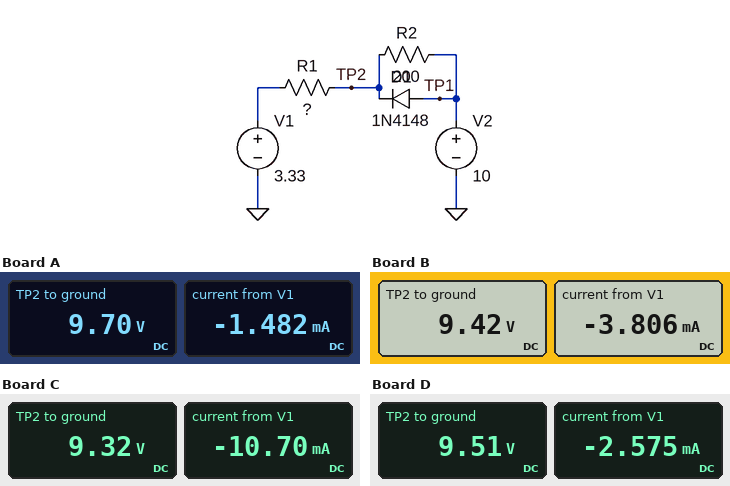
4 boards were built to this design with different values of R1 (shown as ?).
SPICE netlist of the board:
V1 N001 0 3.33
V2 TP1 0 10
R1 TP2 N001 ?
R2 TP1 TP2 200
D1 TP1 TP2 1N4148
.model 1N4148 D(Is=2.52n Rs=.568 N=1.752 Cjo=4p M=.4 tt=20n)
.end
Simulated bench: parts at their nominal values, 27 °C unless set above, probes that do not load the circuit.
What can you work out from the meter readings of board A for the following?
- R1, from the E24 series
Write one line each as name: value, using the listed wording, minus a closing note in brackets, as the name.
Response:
R1, from the E24 series: 4.3 kΩ
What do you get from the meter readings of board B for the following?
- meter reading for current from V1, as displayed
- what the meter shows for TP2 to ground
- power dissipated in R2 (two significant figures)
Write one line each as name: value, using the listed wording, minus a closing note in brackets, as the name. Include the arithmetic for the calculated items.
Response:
meter reading for current from V1, as displayed: -3.806 mA
what the meter shows for TP2 to ground: 9.42 V
power dissipated in R2: (10 V - 9.42 V)^2 / 200 Ω = 1.7 mW
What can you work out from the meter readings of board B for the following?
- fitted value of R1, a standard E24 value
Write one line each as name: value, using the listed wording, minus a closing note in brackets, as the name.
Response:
fitted value of R1, a standard E24 value: 1.6 kΩ
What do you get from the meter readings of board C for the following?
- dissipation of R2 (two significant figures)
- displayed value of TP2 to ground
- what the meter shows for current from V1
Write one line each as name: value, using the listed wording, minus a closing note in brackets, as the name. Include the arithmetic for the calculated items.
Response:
dissipation of R2: (10 V - 9.32 V)^2 / 200 Ω = 2.3 mW
displayed value of TP2 to ground: 9.32 V
what the meter shows for current from V1: -10.70 mA
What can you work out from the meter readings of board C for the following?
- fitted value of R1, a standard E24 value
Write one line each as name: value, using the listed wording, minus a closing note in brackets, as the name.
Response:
fitted value of R1, a standard E24 value: 560 Ω
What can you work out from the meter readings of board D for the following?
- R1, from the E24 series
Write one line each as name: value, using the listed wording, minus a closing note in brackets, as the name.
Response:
R1, from the E24 series: 2.4 kΩ
